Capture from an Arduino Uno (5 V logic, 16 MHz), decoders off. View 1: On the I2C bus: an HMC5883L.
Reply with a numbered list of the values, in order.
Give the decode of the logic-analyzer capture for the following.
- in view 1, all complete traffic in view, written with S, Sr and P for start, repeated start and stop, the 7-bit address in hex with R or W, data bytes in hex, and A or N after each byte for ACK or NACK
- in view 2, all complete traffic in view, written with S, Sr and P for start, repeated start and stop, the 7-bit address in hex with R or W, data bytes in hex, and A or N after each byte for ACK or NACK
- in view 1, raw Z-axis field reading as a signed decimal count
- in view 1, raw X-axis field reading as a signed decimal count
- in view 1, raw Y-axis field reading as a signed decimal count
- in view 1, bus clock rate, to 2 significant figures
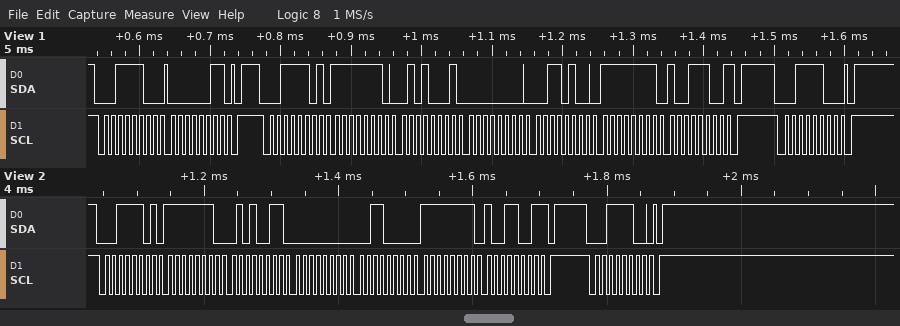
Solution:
1. S 1EW A 03 A P S 1ER A FE A 51 A 00 A 34 A FF A 9C N P S 1EW A P
2. S 1ER A FE A 53 A 00 A 30 A FF A 99 N P S 1EW A P
3. 52
4. -431
5. -100
6. 100 kHz
